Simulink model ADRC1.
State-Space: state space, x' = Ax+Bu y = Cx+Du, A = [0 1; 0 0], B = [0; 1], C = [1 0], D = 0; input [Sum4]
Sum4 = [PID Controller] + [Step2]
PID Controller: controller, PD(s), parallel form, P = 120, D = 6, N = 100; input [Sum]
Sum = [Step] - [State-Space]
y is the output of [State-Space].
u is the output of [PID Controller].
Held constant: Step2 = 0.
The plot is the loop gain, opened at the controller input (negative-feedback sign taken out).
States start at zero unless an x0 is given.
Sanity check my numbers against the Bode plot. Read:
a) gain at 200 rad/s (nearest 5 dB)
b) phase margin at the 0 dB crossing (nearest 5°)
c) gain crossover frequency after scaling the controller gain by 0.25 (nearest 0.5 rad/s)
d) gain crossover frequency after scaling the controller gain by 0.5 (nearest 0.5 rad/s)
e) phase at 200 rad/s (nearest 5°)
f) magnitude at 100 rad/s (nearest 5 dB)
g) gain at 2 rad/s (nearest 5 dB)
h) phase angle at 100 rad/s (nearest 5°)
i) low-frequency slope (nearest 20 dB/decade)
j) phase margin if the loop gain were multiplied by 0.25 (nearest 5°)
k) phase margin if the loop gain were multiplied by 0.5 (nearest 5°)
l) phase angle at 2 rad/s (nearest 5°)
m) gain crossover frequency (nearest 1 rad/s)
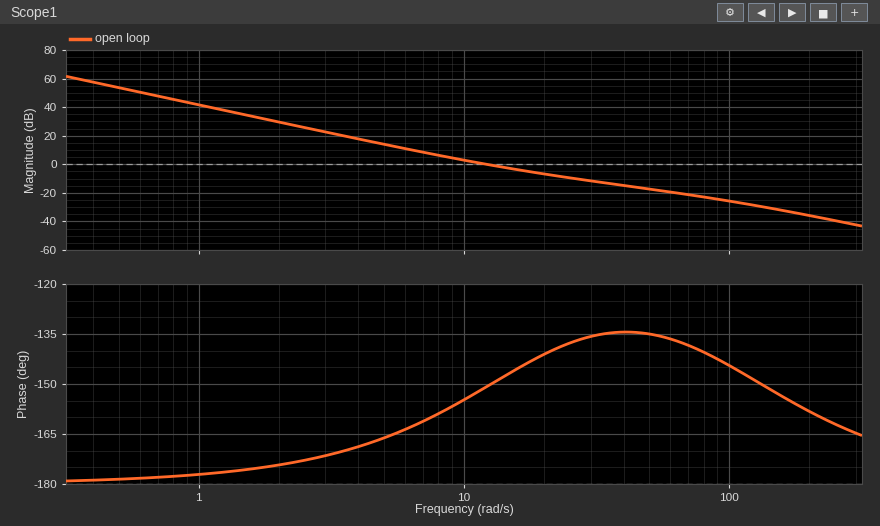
-35 dB
30°
5.5 rad/s
8.0 rad/s
-160°
-25 dB
30 dB
-145°
-40 dB/decade
15°
20°
-175°
12 rad/s
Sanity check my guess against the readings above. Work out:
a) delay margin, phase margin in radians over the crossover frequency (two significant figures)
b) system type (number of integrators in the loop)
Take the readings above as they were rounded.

0.044 s
2
